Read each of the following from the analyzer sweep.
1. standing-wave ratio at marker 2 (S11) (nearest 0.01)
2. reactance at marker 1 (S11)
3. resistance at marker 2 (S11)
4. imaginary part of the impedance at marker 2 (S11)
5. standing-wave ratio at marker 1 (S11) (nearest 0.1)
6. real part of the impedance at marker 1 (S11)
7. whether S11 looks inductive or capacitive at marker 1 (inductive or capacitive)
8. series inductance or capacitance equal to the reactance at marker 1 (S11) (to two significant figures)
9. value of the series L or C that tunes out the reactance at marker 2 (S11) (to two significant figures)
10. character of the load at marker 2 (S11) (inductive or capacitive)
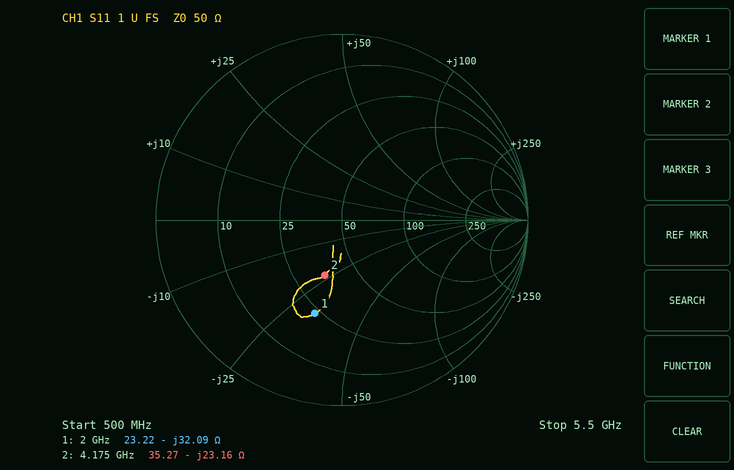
1.90
-32.09 Ω
35.27 Ω
-23.16 Ω
3.2
23.22 Ω
capacitive
2.5 pF
880 pH
capacitive
